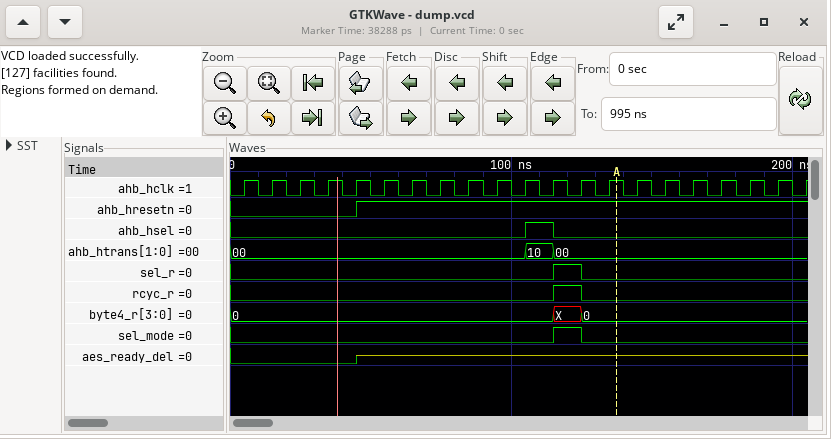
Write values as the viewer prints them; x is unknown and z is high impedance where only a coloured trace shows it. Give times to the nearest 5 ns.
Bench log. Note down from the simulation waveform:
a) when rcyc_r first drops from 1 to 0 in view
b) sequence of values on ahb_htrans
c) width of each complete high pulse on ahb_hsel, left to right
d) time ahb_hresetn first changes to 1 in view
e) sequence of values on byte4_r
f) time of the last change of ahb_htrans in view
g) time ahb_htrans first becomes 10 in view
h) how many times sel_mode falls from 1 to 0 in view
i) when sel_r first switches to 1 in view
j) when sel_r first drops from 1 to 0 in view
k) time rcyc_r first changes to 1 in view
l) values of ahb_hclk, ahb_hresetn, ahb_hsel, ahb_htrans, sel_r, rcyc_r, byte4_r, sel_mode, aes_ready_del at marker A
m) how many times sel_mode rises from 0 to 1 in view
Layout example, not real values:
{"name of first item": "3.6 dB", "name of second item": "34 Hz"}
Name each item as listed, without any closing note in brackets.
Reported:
{"when rcyc_r first drops from 1 to 0 in view": "125 ns", "sequence of values on ahb_htrans": "00, 10, 00", "width of each complete high pulse on ahb_hsel, left to right": "10 ns", "time ahb_hresetn first changes to 1 in view": "45 ns", "sequence of values on byte4_r": "0, X, 0", "time of the last change of ahb_htrans in view": "115 ns", "time ahb_htrans first becomes 10 in view": "105 ns", "how many times sel_mode falls from 1 to 0 in view": "1", "when sel_r first switches to 1 in view": "115 ns", "when sel_r first drops from 1 to 0 in view": "125 ns", "time rcyc_r first changes to 1 in view": "115 ns", "values of ahb_hclk, ahb_hresetn, ahb_hsel, ahb_htrans, sel_r, rcyc_r, byte4_r, sel_mode, aes_ready_del at marker A": "ahb_hclk=1, ahb_hresetn=1, ahb_hsel=0, ahb_htrans=00, sel_r=0, rcyc_r=0, byte4_r=0, sel_mode=0, aes_ready_del=z", "how many times sel_mode rises from 0 to 1 in view": "1"}
